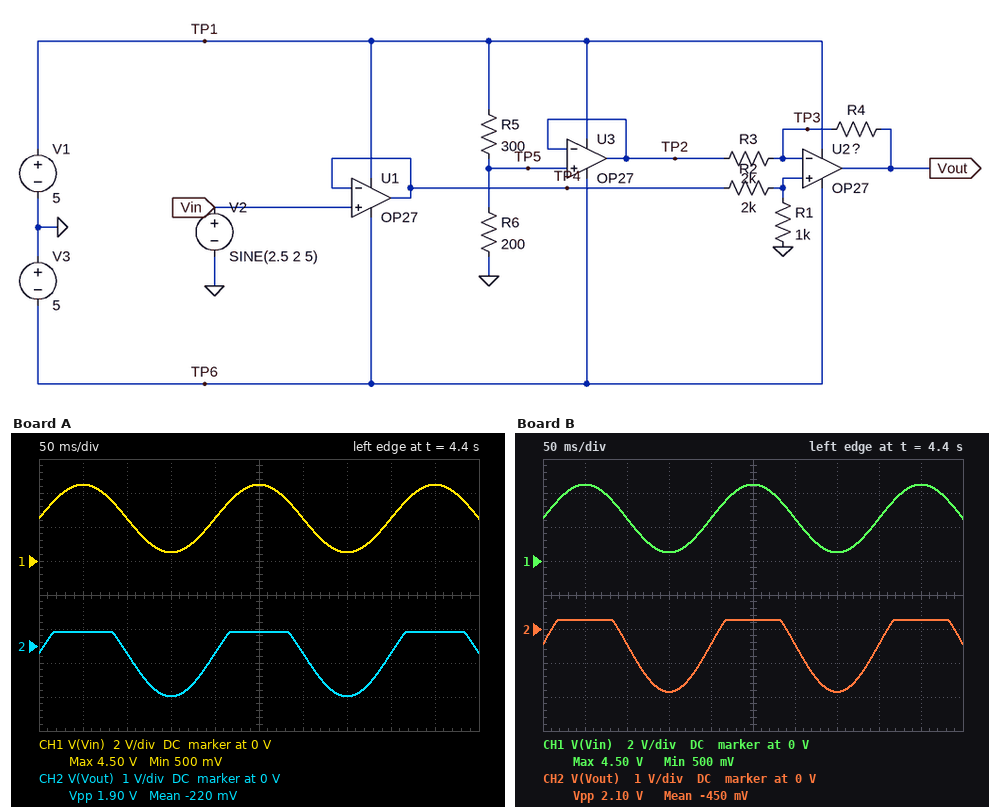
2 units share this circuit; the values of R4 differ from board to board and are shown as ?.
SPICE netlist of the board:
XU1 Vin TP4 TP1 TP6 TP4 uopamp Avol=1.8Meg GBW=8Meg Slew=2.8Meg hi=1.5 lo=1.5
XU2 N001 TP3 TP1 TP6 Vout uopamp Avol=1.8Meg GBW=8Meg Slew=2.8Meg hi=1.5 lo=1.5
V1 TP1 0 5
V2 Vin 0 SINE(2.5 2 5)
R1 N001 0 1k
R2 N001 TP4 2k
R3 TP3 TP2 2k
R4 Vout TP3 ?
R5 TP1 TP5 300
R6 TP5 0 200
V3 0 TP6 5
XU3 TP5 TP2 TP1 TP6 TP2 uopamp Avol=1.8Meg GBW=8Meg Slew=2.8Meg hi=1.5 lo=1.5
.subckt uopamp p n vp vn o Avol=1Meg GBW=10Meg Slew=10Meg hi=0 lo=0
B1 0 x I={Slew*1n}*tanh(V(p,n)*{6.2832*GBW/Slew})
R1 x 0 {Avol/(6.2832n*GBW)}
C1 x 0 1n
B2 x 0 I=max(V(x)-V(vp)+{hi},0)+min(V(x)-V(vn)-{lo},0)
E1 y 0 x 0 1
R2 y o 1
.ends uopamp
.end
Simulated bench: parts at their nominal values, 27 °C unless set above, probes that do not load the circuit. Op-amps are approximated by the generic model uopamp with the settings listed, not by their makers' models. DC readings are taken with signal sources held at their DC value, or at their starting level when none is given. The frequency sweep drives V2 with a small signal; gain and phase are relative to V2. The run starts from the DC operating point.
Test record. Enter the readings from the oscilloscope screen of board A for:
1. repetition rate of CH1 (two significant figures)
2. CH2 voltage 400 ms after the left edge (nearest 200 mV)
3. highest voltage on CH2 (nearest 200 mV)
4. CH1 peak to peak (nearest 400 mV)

5.0 Hz
-200 mV
400 mV
4.0 V
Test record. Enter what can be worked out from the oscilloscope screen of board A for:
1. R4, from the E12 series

1.8 kΩ
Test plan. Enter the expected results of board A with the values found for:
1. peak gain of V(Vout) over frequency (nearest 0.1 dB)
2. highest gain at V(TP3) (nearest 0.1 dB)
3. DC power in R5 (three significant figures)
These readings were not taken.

-4.0 dB
-9.5 dB
30.0 mW
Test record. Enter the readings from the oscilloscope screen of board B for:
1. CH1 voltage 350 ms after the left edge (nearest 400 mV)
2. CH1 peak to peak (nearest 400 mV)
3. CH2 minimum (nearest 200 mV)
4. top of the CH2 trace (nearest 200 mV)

400 mV
4.0 V
-1.8 V
200 mV
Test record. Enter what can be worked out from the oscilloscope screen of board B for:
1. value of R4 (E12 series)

2.2 kΩ
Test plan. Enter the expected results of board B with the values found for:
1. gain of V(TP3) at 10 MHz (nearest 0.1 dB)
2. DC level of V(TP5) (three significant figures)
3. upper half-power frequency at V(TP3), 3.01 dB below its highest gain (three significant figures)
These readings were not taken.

-22.6 dB
2.00 V
3.23 MHz
